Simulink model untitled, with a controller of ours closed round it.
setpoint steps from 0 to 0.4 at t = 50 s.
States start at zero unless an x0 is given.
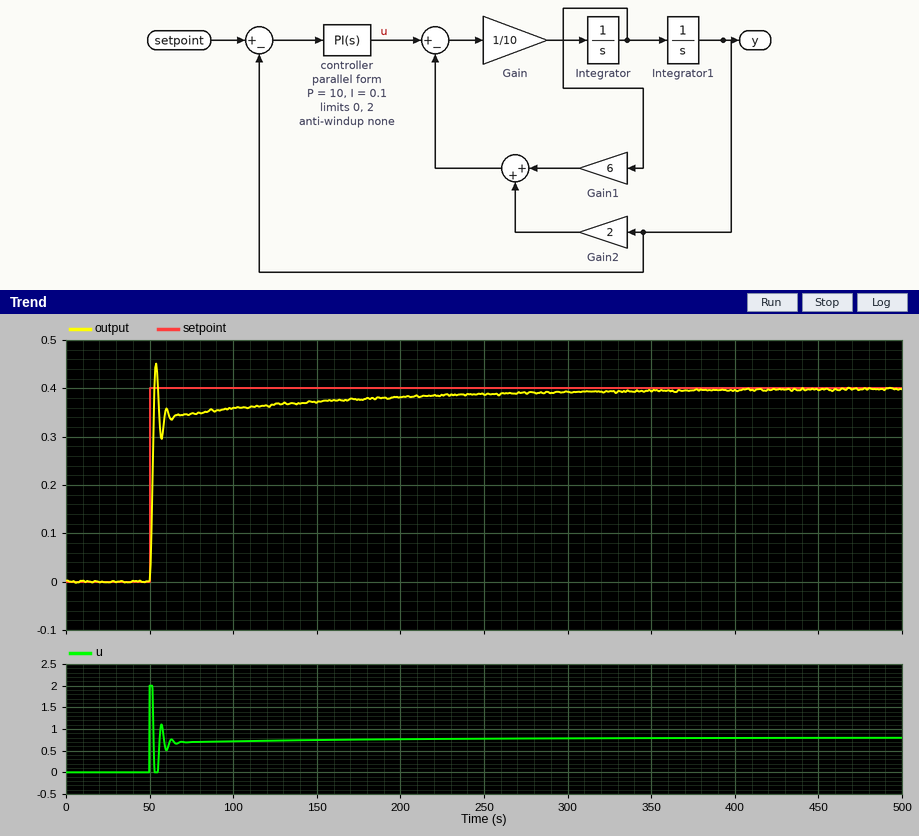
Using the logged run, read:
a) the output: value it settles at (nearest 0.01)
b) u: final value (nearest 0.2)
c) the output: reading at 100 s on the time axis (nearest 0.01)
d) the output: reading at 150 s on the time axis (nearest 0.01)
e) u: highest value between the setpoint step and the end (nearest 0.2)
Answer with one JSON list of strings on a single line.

["0.40", "0.8", "0.36", "0.37", "2.0"]
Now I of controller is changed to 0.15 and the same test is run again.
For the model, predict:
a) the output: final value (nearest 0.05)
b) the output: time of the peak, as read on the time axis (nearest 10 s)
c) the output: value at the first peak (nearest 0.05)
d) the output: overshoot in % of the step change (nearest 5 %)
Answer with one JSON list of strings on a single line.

["0.40", "50 s", "0.45", "15 %"]
